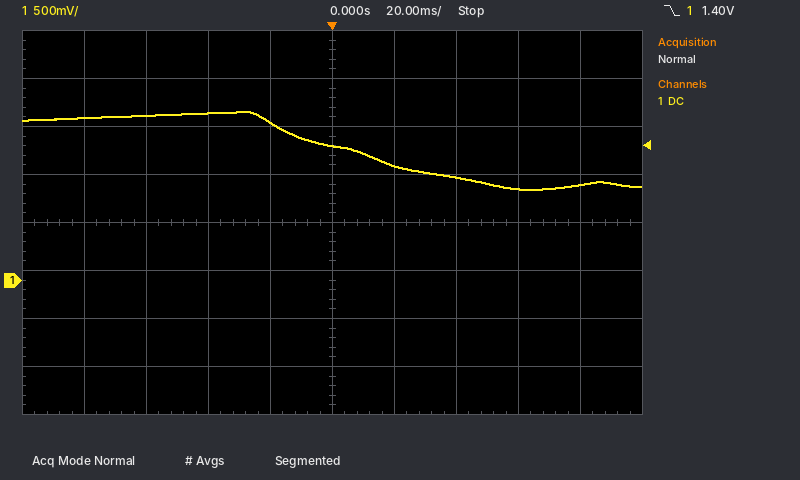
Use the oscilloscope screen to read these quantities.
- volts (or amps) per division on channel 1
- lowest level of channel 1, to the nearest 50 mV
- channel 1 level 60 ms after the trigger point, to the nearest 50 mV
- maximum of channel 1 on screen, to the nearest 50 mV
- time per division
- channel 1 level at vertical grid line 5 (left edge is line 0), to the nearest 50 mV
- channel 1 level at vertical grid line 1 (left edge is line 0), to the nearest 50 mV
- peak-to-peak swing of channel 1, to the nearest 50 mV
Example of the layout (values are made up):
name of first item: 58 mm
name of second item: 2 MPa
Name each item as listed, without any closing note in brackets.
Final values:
volts (or amps) per division on channel 1: 500 mV
lowest level of channel 1, to the nearest 50 mV: 950 mV
channel 1 level 60 ms after the trigger point, to the nearest 50 mV: 950 mV
maximum of channel 1 on screen, to the nearest 50 mV: 1.75 V
time per division: 20 ms
channel 1 level at vertical grid line 5 (left edge is line 0), to the nearest 50 mV: 1.40 V
channel 1 level at vertical grid line 1 (left edge is line 0), to the nearest 50 mV: 1.70 V
peak-to-peak swing of channel 1, to the nearest 50 mV: 800 mV
